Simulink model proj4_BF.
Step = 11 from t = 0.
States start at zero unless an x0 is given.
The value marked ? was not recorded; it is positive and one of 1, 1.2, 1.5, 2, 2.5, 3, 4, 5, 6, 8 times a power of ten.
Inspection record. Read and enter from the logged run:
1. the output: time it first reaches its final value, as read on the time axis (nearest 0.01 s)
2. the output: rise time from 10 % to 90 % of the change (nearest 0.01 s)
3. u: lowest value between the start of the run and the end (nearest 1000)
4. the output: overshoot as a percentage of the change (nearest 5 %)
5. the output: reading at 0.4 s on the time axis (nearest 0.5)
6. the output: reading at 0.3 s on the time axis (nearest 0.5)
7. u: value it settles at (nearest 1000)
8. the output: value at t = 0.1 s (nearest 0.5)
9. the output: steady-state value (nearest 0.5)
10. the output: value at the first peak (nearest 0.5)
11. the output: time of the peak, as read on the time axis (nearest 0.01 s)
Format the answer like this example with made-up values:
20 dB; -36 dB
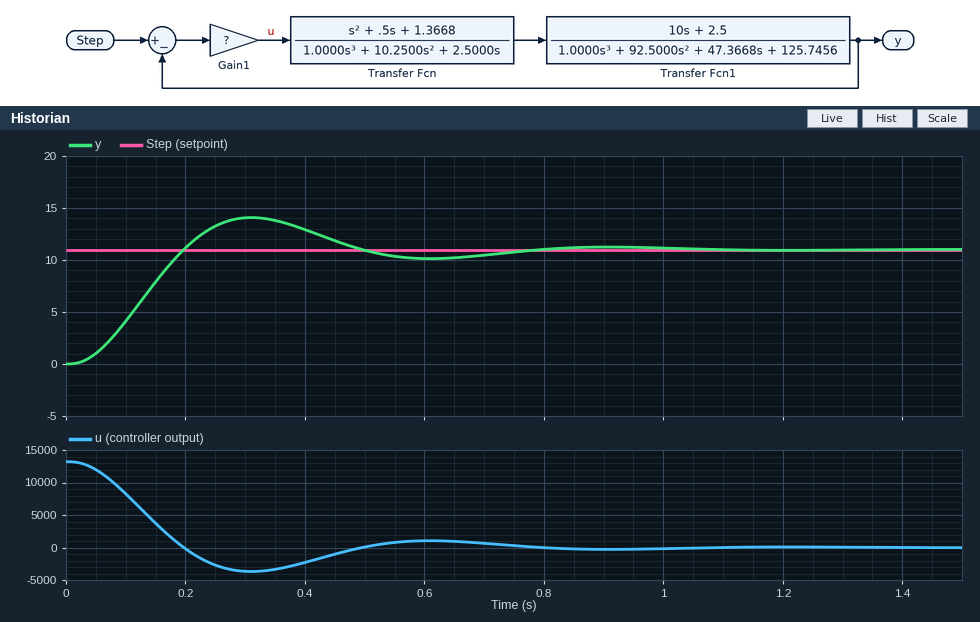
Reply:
0.20 s; 0.13 s; -4000; 30 %; 13.0; 14.0; 0; 4.0; 11.0; 14.0; 0.31 s
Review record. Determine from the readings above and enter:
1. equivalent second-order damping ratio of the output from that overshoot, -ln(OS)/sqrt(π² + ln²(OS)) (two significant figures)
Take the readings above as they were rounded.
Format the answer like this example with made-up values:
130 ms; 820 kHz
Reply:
0.36
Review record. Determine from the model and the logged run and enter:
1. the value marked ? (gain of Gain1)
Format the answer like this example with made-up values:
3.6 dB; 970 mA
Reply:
1200
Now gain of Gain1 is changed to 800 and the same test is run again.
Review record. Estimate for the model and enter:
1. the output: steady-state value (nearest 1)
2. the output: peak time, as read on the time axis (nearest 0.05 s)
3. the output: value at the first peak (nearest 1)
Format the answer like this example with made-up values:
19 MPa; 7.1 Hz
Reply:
11; 0.40 s; 13
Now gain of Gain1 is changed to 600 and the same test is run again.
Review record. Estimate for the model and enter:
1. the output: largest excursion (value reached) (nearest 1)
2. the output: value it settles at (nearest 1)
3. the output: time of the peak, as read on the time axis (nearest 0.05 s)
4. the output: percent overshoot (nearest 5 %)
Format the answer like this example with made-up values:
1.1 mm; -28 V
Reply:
12; 11; 0.50 s; 10 %
